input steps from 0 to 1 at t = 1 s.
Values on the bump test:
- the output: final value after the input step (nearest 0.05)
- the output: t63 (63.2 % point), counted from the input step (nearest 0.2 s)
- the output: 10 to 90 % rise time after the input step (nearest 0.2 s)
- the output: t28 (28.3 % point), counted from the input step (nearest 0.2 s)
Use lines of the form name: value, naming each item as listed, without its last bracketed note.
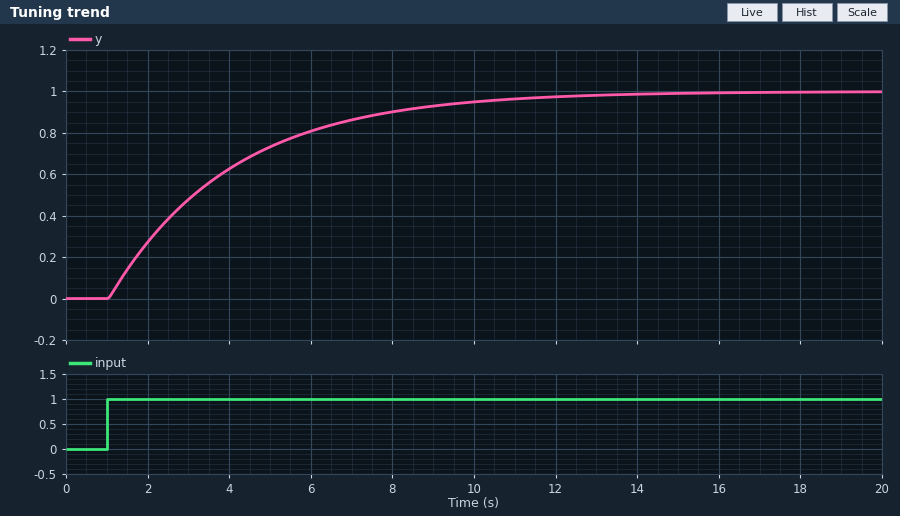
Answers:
the output: final value after the input step: 1.00
the output: t63 (63.2 % point), counted from the input step: 3.0 s
the output: 10 to 90 % rise time after the input step: 6.6 s
the output: t28 (28.3 % point), counted from the input step: 1.0 s
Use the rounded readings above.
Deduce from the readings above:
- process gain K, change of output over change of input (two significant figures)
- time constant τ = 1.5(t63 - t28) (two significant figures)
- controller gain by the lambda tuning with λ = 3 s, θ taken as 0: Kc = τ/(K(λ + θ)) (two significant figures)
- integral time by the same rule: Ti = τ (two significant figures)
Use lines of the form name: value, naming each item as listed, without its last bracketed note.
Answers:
process gain K, change of output over change of input: 1.0
time constant τ = 1.5(t63 - t28): 3.0 s
controller gain by the lambda tuning with λ = 3 s, θ taken as 0: Kc = τ/(K(λ + θ)): 1.0
integral time by the same rule: Ti = τ: 3.0 s
